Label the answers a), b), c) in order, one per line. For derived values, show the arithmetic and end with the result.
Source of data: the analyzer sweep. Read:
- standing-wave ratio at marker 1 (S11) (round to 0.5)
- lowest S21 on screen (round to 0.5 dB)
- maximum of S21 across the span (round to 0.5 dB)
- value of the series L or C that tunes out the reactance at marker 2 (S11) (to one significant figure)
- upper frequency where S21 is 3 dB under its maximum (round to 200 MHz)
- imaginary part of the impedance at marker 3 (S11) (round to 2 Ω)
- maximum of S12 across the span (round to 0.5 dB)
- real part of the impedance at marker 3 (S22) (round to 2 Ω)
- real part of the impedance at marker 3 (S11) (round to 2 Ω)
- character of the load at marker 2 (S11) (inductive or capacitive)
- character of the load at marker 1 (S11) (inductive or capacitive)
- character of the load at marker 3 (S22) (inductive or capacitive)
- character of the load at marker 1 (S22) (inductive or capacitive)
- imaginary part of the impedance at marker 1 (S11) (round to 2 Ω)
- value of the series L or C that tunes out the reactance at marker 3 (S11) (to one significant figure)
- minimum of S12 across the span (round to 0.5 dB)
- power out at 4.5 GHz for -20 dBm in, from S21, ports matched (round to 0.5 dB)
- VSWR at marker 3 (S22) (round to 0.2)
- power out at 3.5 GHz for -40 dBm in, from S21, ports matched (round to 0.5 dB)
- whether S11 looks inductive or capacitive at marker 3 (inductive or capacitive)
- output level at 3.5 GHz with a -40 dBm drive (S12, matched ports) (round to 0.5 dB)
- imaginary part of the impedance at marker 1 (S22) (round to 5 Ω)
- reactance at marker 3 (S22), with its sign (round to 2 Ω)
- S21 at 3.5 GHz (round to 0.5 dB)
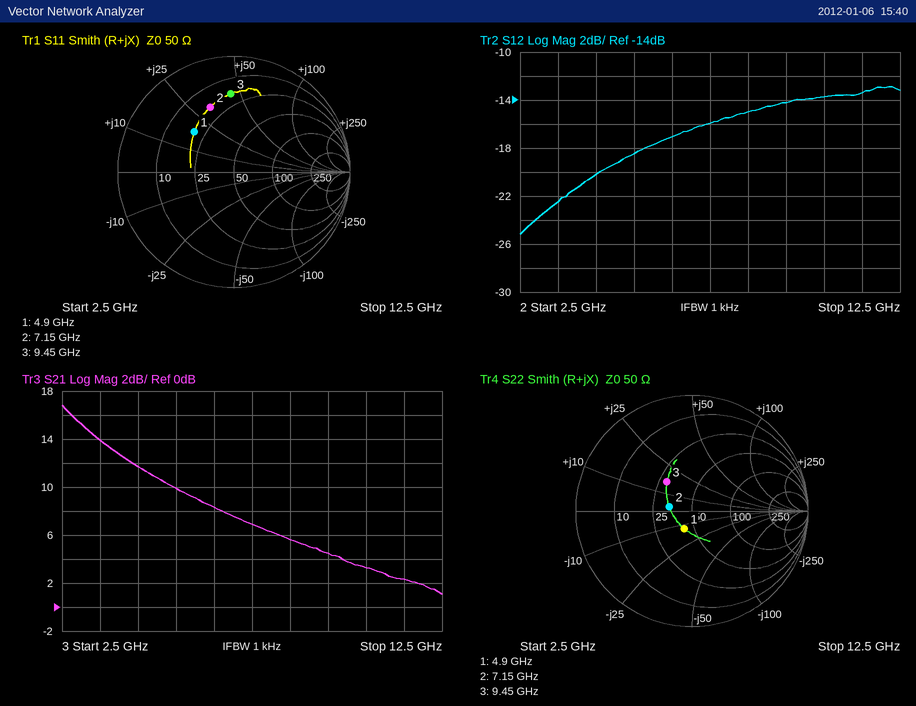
a) 3.0
b) 1.0 dB
c) 17.0 dB
d) C = 1/(2π × 7.15 GHz × 32 Ω) ≈ 696 fF, so 700 fF to one significant figure
e) 3.6 GHz
f) +44 Ω
g) -13.0 dB
h) 28 Ω
i) 18 Ω
j) inductive
k) inductive
l) inductive
m) capacitive
n) +18 Ω
o) C = 1/(2π × 9.45 GHz × 44 Ω) ≈ 383 fF, so 400 fF to one significant figure
p) -25.0 dB
q) -20 dBm + (11.5 dB) = -8.5 dBm
r) 2.0
s) -40 dBm + (14.0 dB) = -26.0 dBm
t) inductive
u) -40 dBm + (-22.5 dB) = -62.5 dBm
v) -15 Ω
w) +16 Ω
x) 14.0 dB
